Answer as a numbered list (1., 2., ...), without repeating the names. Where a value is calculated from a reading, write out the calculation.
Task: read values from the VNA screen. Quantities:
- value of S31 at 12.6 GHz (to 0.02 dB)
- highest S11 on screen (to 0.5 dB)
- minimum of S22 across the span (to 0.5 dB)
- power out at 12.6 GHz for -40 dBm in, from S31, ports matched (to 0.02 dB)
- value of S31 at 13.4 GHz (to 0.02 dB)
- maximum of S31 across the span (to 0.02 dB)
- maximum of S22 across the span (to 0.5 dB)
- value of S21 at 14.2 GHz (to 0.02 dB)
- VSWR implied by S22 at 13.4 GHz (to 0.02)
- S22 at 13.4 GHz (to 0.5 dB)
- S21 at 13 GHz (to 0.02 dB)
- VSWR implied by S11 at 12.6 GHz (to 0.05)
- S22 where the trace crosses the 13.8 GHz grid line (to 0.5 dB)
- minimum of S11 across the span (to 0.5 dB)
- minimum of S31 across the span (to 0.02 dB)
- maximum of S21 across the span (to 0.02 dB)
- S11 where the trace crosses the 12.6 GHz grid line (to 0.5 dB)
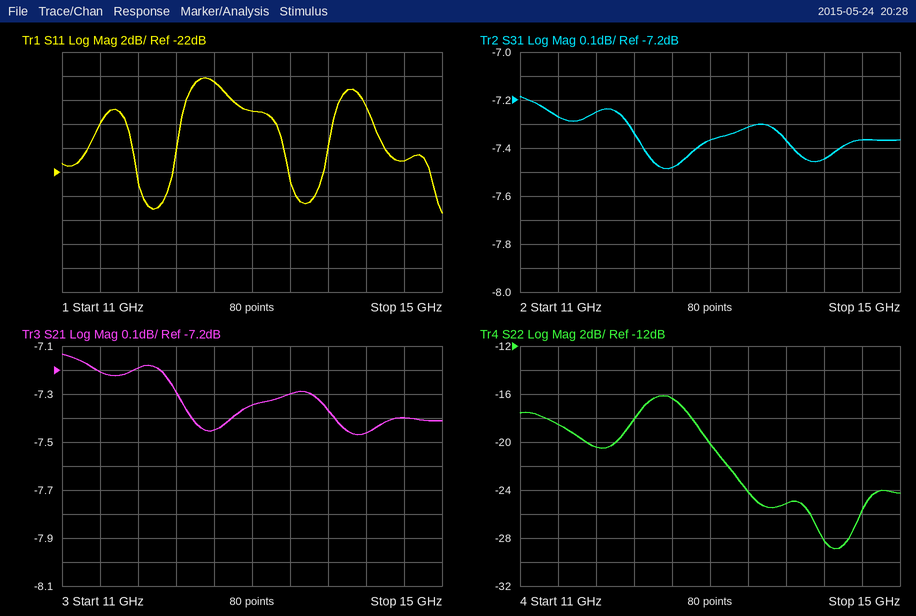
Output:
1. -7.48 dB
2. -14.0 dB
3. -29.0 dB
4. -40 dBm + (-7.48 dB) = -47.48 dBm
5. -7.32 dB
6. -7.18 dB
7. -16.0 dB
8. -7.46 dB
9. |Γ| = 10^(-24/20) = 0.0631; VSWR = (1 + 0.0631)/(1 − 0.0631) ≈ 1.13, so 1.14 to the nearest 0.02
10. -24.0 dB
11. -7.34 dB
12. |Γ| = 10^(-14.5/20) = 0.1884; VSWR = (1 + 0.1884)/(1 − 0.1884) ≈ 1.46, so 1.45 to the nearest 0.05
13. -25.0 dB
14. -25.5 dB
15. -7.48 dB
16. -7.14 dB
17. -14.5 dB
